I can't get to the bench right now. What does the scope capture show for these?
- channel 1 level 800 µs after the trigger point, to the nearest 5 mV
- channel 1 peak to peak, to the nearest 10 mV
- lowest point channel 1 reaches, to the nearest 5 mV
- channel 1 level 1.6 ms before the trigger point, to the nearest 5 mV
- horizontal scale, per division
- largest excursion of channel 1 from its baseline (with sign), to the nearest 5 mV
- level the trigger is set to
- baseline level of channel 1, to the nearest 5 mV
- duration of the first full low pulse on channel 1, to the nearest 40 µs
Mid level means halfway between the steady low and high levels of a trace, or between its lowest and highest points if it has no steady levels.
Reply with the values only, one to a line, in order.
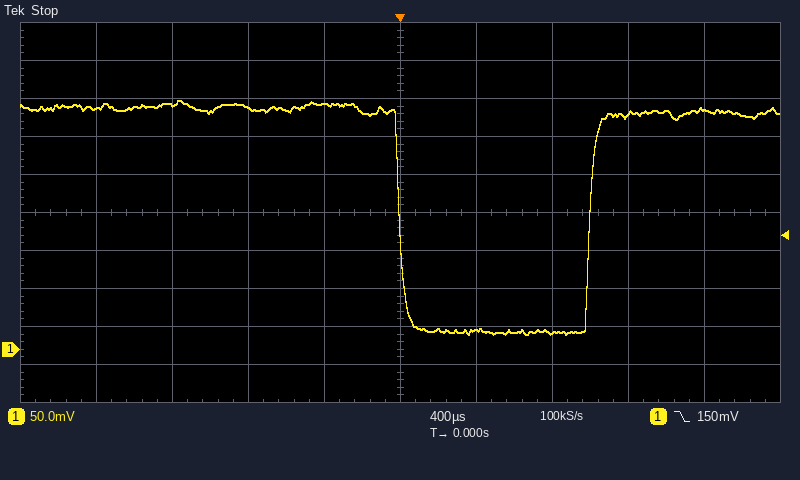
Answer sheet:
20 mV
310 mV
20 mV
315 mV
400 µs
-295 mV
150 mV
315 mV
1.00 ms
